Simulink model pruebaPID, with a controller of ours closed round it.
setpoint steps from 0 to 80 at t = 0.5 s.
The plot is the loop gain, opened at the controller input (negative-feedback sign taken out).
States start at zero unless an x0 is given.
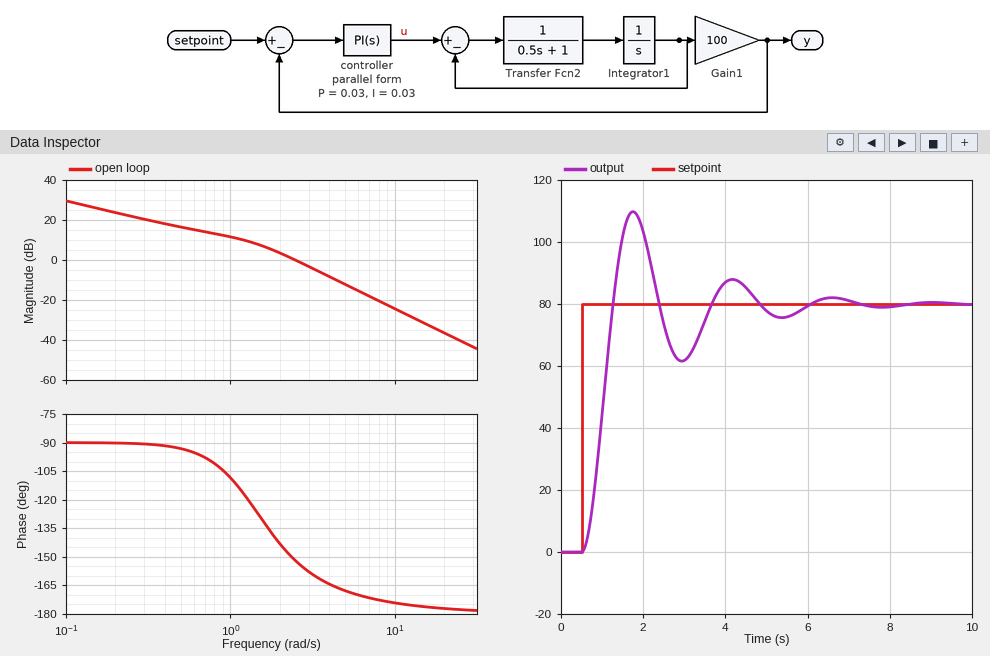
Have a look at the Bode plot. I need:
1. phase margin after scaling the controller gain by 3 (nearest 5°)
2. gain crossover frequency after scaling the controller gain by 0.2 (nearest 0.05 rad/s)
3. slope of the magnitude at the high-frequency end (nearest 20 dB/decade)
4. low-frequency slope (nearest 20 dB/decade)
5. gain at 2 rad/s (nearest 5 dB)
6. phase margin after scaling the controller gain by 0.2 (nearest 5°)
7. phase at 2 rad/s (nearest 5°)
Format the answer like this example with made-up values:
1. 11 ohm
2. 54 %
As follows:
1. 15°
2. 0.70 rad/s
3. -40 dB/decade
4. -20 dB/decade
5. 5 dB
6. 80°
7. -145°
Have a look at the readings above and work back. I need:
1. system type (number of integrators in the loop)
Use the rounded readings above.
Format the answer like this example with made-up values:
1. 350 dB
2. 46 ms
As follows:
1. 1
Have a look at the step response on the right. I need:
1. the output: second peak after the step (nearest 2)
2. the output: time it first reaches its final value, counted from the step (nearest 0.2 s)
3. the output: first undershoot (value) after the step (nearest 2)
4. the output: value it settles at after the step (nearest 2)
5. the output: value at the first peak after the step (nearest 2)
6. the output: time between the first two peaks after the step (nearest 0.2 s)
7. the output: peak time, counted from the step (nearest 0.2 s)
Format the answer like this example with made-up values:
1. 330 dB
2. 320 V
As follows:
1. 88
2. 0.8 s
3. 62
4. 80
5. 110
6. 2.4 s
7. 1.2 s
